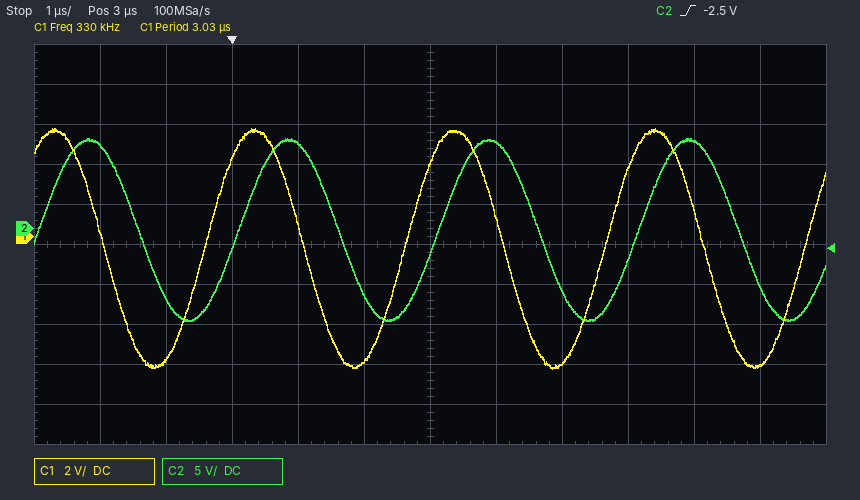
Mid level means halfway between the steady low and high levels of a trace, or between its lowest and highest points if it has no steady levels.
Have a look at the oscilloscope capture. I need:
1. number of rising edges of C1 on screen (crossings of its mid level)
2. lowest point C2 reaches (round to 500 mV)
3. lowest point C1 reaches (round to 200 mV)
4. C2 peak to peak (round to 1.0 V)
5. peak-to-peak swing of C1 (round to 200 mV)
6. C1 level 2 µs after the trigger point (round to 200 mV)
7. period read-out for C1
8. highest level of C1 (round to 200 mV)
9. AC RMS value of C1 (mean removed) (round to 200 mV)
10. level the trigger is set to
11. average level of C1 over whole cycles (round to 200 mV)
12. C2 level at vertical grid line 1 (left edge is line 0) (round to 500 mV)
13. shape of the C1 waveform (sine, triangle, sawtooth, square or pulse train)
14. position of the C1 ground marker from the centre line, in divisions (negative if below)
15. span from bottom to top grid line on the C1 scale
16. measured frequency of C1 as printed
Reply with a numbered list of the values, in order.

1. 4
2. -11.5 V
3. -6.6 V
4. 23.0 V
5. 12.0 V
6. -6.2 V
7. 3.03 µs
8. 5.4 V
9. 4.2 V
10. -2.5 V
11. -600 mV
12. 10.5 V
13. sine
14. +0.2 div
15. 20 V
16. 330 kHz
